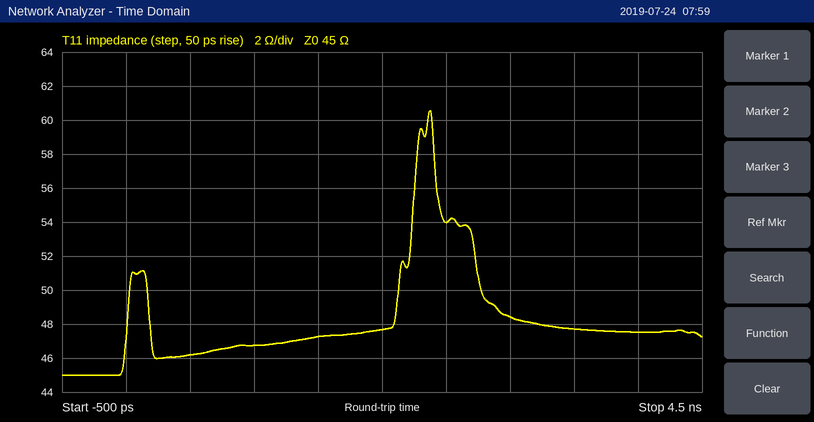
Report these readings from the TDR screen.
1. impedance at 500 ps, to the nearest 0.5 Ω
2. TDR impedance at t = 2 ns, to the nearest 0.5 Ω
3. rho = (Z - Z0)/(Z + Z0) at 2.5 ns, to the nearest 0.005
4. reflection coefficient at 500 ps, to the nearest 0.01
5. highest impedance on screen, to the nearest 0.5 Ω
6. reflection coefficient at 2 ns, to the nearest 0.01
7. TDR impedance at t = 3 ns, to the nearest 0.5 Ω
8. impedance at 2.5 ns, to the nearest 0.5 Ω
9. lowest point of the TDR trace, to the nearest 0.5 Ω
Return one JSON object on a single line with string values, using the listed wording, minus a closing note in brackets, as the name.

{"impedance at 500 ps, to the nearest 0.5 Ω": "46.0 Ω", "TDR impedance at t = 2 ns, to the nearest 0.5 Ω": "47.5 Ω", "rho = (Z - Z0)/(Z + Z0) at 2.5 ns, to the nearest 0.005": "+0.090", "reflection coefficient at 500 ps, to the nearest 0.01": "+0.01", "highest impedance on screen, to the nearest 0.5 Ω": "60.5 Ω", "reflection coefficient at 2 ns, to the nearest 0.01": "+0.03", "TDR impedance at t = 3 ns, to the nearest 0.5 Ω": "48.5 Ω", "impedance at 2.5 ns, to the nearest 0.5 Ω": "54.0 Ω", "lowest point of the TDR trace, to the nearest 0.5 Ω": "45.0 Ω"}
